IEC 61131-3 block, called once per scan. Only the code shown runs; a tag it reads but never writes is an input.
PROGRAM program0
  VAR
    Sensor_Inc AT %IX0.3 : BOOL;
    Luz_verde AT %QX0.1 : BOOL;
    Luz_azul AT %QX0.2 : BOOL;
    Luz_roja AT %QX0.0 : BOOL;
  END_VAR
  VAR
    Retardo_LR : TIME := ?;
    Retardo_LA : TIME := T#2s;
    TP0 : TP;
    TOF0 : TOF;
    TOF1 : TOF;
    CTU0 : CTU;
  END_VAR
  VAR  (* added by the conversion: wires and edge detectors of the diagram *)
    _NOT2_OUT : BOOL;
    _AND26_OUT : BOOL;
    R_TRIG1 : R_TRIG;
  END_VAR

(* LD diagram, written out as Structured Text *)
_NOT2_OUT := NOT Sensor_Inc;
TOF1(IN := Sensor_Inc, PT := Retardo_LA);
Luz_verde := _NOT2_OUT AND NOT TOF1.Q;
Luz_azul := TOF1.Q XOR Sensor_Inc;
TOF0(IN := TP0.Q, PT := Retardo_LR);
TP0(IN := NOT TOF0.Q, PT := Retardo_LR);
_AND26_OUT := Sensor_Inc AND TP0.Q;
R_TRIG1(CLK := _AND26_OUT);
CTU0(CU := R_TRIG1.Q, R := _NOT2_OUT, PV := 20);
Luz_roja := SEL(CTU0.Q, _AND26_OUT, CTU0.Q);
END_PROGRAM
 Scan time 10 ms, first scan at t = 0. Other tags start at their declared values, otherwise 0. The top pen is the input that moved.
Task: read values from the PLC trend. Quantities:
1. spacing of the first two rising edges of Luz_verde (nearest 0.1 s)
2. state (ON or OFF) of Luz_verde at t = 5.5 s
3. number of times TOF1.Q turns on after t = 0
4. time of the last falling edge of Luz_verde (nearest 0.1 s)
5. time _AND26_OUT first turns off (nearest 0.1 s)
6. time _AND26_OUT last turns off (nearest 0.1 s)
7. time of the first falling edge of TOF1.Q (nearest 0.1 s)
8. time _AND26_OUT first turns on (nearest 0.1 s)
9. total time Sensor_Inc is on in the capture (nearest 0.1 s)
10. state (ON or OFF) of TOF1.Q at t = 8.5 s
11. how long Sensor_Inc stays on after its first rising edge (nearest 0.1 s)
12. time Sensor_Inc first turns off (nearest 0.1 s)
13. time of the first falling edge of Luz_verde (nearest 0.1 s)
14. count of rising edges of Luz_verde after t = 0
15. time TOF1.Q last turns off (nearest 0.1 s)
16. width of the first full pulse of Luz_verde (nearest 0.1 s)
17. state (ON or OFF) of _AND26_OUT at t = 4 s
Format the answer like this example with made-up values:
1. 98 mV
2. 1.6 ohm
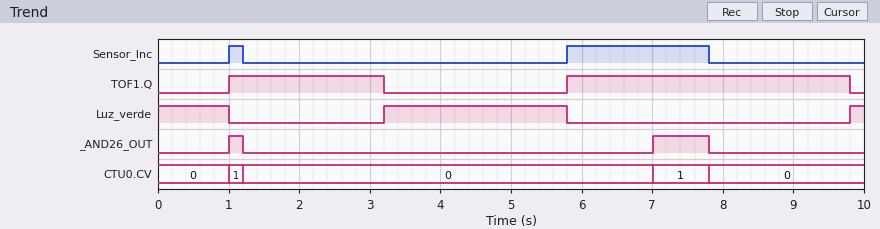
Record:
1. 6.6 s
2. ON
3. 2
4. 5.8 s
5. 1.2 s
6. 7.8 s
7. 3.2 s
8. 1.0 s
9. 2.2 s
10. ON
11. 0.2 s
12. 1.2 s
13. 1.0 s
14. 2
15. 9.8 s
16. 2.6 s
17. OFF
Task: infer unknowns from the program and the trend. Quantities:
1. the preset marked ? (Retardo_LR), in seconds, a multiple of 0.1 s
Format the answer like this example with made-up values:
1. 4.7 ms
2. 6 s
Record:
1. 3.5 s
